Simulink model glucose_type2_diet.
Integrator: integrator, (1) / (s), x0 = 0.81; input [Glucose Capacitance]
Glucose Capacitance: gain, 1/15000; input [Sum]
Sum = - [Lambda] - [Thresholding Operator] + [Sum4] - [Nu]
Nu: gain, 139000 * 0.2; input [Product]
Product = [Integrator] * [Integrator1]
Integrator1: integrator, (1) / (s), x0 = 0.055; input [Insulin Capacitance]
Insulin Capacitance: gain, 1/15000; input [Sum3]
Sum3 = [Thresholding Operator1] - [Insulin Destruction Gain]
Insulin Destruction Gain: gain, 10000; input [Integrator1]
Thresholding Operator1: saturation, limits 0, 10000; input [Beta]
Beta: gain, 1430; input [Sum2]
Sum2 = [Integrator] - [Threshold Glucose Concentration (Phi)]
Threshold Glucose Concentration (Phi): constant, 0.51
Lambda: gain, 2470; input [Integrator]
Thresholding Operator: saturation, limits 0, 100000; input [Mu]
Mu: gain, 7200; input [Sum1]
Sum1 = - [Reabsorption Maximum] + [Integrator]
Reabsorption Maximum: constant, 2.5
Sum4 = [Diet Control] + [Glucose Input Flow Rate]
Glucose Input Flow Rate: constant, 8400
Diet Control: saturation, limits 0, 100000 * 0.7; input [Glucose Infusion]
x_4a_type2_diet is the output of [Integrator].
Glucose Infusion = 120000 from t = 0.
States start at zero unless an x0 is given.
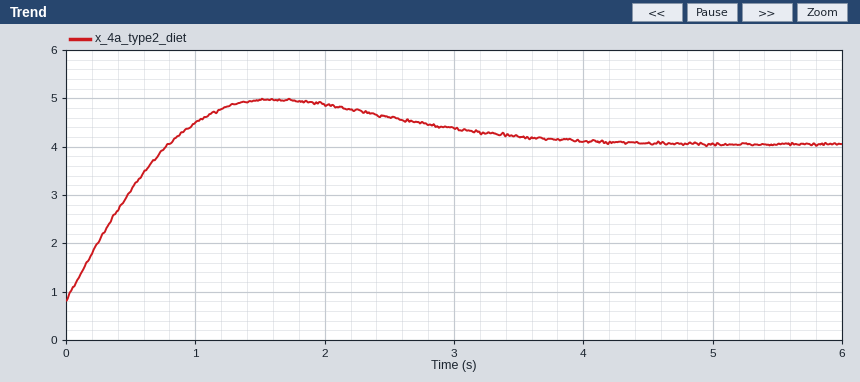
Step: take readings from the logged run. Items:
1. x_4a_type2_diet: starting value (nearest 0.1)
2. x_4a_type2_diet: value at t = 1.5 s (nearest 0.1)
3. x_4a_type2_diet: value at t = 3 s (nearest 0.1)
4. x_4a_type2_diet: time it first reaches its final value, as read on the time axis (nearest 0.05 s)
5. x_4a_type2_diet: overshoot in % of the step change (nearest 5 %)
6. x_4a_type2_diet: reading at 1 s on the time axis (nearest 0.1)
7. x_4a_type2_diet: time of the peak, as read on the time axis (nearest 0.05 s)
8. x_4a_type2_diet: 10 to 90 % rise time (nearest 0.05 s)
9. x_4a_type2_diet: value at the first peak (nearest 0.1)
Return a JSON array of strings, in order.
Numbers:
["0.8", "5.0", "4.4", "0.80 s", "30 %", "4.5", "1.60 s", "0.60 s", "5.0"]
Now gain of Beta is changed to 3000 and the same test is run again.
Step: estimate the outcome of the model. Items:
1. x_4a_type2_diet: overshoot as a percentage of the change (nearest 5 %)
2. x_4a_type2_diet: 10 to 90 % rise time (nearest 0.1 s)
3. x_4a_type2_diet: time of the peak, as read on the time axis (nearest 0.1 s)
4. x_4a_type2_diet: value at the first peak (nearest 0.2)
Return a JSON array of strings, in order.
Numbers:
["50 %", "0.4 s", "1.2 s", "4.2"]
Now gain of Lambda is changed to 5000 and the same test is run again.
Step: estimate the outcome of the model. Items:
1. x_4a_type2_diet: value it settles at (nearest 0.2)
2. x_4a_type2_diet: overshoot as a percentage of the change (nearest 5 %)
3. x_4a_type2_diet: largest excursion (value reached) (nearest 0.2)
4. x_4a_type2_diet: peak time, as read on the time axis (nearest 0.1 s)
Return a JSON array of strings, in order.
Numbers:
["3.8", "25 %", "4.6", "1.6 s"]
